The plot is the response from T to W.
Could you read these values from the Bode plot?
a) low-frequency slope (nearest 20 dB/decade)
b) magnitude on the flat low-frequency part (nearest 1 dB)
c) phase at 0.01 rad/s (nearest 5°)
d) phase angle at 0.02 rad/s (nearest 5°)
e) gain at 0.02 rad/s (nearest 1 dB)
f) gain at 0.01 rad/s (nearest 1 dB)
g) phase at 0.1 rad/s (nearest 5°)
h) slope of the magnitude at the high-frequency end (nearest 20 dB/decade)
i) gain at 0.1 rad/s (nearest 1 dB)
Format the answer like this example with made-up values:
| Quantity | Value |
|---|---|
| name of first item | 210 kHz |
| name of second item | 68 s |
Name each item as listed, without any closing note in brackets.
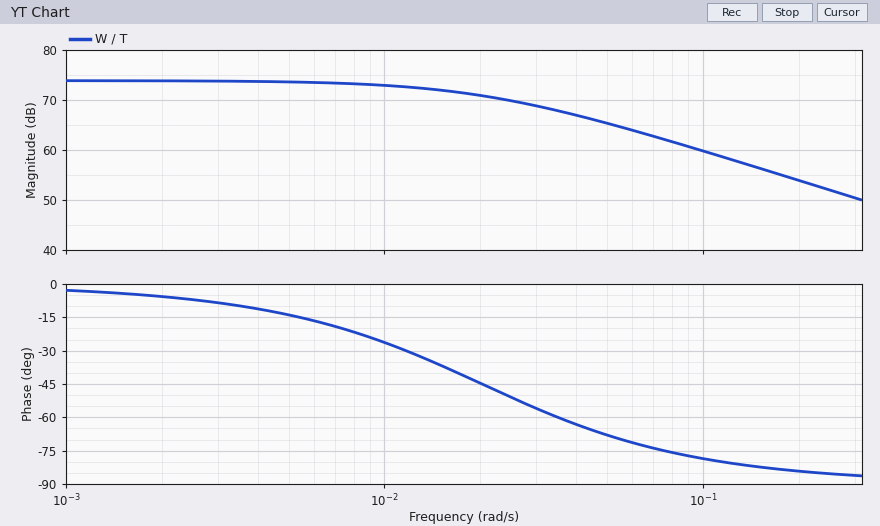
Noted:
| Quantity | Value |
|---|---|
| low-frequency slope | 0 dB/decade |
| magnitude on the flat low-frequency part | 74 dB |
| phase at 0.01 rad/s | -25° |
| phase angle at 0.02 rad/s | -45° |
| gain at 0.02 rad/s | 71 dB |
| gain at 0.01 rad/s | 73 dB |
| phase at 0.1 rad/s | -80° |
| slope of the magnitude at the high-frequency end | -20 dB/decade |
| gain at 0.1 rad/s | 60 dB |
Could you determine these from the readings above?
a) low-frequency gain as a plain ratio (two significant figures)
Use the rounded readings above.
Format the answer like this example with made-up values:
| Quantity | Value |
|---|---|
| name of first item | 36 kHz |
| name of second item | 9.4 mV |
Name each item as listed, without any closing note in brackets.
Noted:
| Quantity | Value |
|---|---|
| low-frequency gain as a plain ratio | 5000 |
